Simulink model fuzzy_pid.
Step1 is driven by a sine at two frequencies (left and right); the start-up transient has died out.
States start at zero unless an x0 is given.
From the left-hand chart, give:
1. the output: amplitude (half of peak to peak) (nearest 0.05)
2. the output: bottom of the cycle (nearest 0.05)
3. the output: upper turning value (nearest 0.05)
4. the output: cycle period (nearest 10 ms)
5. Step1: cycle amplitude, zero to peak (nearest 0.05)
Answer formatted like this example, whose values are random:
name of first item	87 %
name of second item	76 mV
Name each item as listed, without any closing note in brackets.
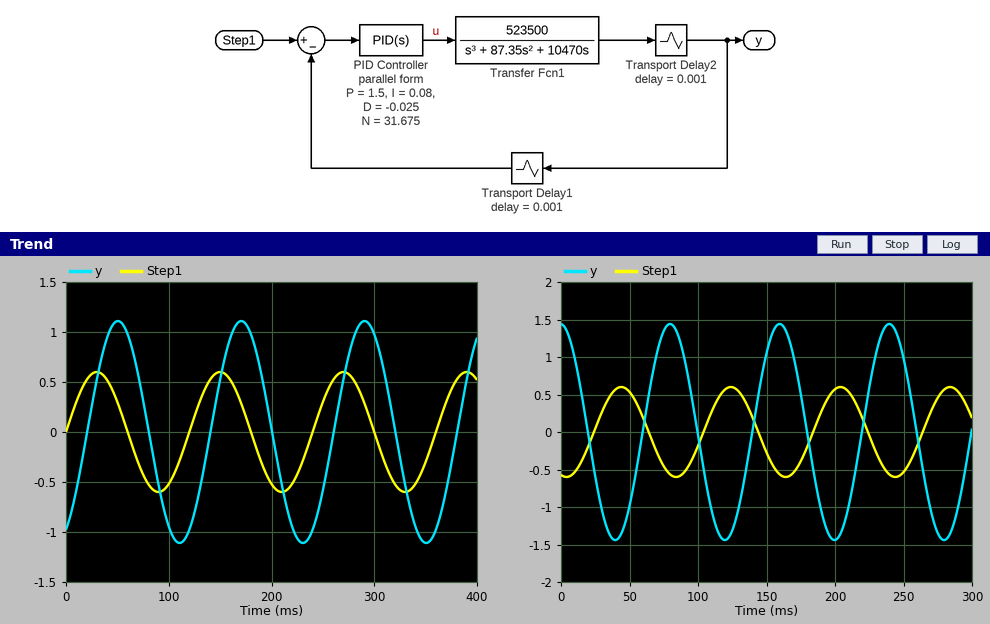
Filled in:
the output: amplitude (half of peak to peak)	1.10
the output: bottom of the cycle	-1.10
the output: upper turning value	1.10
the output: cycle period	120 ms
Step1: cycle amplitude, zero to peak	0.60
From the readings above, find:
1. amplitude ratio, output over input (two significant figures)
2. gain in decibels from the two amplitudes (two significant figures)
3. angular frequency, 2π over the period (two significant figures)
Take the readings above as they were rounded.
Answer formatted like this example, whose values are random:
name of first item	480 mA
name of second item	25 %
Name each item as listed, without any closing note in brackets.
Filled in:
amplitude ratio, output over input	1.8
gain in decibels from the two amplitudes	5.3 dB
angular frequency, 2π over the period	0.052 rad/ms
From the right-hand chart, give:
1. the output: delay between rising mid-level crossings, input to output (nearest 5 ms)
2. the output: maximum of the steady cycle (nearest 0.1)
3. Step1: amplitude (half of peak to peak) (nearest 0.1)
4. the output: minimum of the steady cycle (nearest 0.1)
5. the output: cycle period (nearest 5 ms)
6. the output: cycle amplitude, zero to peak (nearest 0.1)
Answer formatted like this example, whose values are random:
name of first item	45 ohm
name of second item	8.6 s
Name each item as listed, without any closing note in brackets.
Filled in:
the output: delay between rising mid-level crossings, input to output	35 ms
the output: maximum of the steady cycle	1.4
Step1: amplitude (half of peak to peak)	0.6
the output: minimum of the steady cycle	-1.4
the output: cycle period	80 ms
the output: cycle amplitude, zero to peak	1.4
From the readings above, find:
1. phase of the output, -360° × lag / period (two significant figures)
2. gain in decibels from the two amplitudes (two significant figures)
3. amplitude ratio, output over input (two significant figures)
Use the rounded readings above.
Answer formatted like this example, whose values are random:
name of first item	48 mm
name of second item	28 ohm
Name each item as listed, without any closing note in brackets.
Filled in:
phase of the output, -360° × lag / period	-160°
gain in decibels from the two amplitudes	7.4 dB
amplitude ratio, output over input	2.3
